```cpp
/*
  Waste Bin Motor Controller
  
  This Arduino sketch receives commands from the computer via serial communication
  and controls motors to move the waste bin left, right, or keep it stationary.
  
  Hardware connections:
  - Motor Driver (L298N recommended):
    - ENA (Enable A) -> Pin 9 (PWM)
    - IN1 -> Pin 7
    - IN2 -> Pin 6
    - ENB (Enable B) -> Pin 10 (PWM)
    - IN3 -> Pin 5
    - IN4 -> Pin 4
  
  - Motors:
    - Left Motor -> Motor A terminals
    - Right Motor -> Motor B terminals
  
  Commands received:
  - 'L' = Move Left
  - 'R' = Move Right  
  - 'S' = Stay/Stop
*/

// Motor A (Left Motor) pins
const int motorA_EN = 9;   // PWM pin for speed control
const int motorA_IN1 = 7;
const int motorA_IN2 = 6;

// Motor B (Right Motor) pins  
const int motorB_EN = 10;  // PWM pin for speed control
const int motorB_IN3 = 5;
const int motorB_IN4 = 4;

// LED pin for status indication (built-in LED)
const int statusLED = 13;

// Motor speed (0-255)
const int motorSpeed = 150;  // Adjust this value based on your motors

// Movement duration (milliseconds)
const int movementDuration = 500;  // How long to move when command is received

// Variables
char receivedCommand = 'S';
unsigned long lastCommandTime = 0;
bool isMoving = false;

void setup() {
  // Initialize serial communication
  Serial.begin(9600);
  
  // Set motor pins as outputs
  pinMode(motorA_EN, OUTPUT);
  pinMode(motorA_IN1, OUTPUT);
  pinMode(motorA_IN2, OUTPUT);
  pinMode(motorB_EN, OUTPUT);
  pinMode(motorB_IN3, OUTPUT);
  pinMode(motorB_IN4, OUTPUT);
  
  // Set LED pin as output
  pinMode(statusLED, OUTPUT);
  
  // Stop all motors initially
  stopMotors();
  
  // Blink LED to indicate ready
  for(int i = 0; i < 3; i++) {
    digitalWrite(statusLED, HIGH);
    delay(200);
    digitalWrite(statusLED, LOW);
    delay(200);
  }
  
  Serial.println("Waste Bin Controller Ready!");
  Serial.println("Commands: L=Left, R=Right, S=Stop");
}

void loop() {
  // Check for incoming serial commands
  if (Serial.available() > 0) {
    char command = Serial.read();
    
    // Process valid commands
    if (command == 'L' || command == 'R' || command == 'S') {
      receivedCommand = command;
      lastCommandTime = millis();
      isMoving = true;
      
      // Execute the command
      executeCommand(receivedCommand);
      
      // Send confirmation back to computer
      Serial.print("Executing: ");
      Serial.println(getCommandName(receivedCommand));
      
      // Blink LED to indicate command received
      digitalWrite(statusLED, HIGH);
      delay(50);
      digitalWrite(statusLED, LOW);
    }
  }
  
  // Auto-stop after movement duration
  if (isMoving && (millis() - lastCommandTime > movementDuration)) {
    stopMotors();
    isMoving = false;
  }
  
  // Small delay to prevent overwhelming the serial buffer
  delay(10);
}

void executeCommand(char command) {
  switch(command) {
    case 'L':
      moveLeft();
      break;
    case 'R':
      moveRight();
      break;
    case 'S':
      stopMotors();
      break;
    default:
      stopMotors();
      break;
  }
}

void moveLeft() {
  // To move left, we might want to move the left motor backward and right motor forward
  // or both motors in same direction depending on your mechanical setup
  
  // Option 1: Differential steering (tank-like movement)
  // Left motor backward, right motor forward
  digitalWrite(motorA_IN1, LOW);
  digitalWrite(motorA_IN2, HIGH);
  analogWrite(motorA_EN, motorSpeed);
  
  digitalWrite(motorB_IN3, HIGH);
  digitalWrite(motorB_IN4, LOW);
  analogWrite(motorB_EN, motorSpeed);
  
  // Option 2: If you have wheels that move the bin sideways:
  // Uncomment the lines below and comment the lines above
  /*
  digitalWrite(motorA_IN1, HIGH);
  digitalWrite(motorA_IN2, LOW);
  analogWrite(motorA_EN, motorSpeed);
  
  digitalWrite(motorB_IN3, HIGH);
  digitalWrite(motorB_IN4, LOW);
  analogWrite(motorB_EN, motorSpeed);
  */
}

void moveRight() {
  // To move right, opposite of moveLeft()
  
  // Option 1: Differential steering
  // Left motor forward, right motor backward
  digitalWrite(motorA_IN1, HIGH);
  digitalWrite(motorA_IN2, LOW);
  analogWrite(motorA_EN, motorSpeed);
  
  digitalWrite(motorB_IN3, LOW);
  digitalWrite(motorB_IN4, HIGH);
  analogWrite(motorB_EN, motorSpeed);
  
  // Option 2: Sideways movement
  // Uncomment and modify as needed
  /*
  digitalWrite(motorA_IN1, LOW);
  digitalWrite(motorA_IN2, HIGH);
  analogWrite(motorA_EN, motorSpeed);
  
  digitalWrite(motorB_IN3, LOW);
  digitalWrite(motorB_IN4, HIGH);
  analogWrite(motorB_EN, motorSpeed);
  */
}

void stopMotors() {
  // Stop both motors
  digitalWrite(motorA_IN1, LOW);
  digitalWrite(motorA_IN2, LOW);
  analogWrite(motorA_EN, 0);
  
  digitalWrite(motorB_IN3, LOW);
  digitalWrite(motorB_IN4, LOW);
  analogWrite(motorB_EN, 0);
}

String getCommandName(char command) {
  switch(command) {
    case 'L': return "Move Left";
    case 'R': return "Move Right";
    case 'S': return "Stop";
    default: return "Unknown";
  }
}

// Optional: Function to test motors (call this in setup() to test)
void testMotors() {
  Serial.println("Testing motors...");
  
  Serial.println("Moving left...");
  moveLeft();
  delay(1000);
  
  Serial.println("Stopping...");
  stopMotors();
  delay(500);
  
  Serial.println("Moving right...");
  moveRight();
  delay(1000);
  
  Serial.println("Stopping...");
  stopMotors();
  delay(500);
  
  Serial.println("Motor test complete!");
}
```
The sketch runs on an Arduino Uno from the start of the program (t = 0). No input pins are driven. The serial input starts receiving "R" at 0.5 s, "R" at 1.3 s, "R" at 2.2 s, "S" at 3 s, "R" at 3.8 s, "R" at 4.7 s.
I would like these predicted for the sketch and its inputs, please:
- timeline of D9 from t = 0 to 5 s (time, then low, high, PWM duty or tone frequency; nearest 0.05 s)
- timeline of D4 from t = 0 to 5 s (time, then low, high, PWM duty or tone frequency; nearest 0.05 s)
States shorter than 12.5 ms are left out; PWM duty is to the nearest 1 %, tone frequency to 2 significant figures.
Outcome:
0 s low; 1.2 s PWM 59 %; 1.8 s low; 2.2 s PWM 59 %; 2.7 s low; 3.8 s PWM 59 %; 4.3 s low; 4.7 s PWM 59 %
0 s low; 1.2 s high; 1.8 s low; 2.2 s high; 2.7 s low; 3.8 s high; 4.3 s low; 4.7 s high
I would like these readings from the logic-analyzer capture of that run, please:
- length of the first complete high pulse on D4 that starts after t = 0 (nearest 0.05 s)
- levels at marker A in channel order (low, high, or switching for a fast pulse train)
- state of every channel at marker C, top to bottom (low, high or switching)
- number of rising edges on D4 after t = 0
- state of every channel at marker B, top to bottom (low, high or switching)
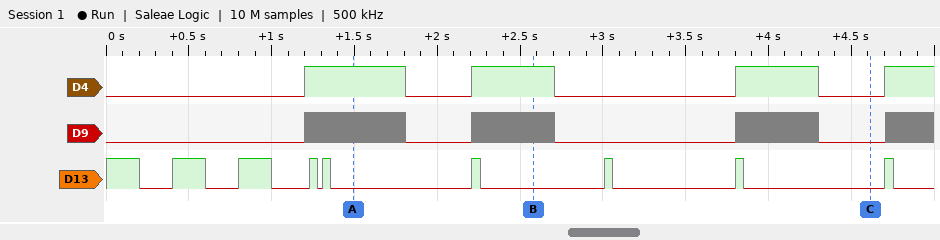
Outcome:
0.60 s
D4 high, D9 switching, D13 low
D4 low, D9 low, D13 low
4
D4 high, D9 switching, D13 low
